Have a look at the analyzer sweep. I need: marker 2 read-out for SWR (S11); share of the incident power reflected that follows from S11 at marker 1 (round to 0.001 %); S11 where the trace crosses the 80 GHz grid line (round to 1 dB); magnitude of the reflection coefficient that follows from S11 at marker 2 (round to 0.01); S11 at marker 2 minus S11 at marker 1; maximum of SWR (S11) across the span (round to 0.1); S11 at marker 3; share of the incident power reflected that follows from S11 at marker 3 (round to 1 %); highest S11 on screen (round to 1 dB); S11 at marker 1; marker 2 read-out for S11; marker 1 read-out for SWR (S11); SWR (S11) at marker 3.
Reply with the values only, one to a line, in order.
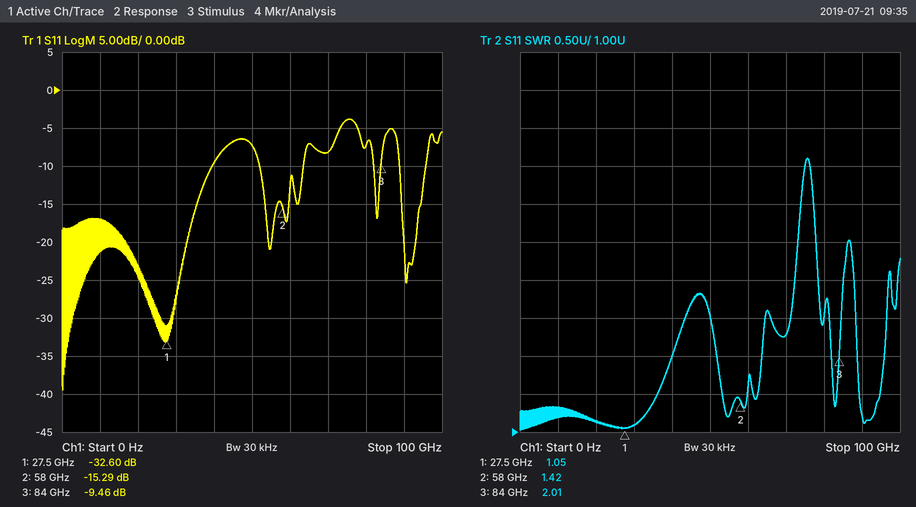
1.42
0.055 %
-7 dB
0.17
17.31 dB
4.6
-9.46 dB
11 %
-4 dB
-32.60 dB
-15.29 dB
1.05
2.01
